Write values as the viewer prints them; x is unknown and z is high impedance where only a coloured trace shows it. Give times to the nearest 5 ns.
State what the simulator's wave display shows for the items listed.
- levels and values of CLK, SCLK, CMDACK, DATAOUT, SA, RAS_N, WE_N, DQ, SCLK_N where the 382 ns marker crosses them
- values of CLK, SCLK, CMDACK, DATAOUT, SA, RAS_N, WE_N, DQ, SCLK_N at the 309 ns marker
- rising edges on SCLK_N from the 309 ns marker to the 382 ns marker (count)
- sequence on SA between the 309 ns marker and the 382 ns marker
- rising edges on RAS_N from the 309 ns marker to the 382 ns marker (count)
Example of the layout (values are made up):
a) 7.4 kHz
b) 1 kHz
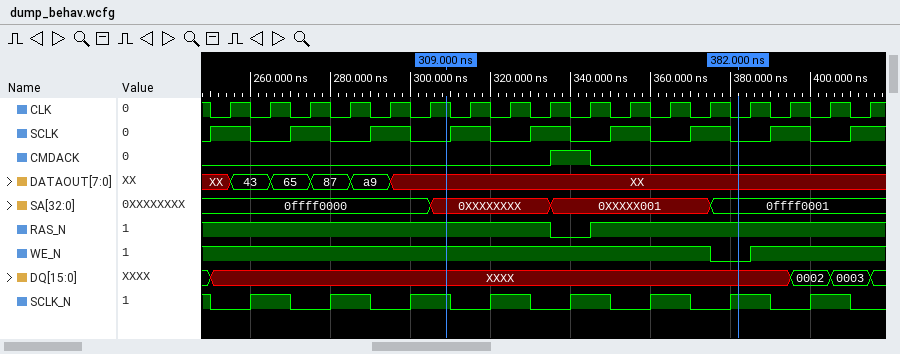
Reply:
a) CLK=0, SCLK=0, CMDACK=0, DATAOUT=XX, SA=0ffff0001, RAS_N=1, WE_N=0, DQ=XXXX, SCLK_N=1
b) CLK=1, SCLK=0, CMDACK=0, DATAOUT=XX, SA=0XXXXXXXX, RAS_N=1, WE_N=1, DQ=XXXX, SCLK_N=1
c) 4
d) 0XXXXXXXX, 0XXXXX001, 0ffff0001
e) 1
